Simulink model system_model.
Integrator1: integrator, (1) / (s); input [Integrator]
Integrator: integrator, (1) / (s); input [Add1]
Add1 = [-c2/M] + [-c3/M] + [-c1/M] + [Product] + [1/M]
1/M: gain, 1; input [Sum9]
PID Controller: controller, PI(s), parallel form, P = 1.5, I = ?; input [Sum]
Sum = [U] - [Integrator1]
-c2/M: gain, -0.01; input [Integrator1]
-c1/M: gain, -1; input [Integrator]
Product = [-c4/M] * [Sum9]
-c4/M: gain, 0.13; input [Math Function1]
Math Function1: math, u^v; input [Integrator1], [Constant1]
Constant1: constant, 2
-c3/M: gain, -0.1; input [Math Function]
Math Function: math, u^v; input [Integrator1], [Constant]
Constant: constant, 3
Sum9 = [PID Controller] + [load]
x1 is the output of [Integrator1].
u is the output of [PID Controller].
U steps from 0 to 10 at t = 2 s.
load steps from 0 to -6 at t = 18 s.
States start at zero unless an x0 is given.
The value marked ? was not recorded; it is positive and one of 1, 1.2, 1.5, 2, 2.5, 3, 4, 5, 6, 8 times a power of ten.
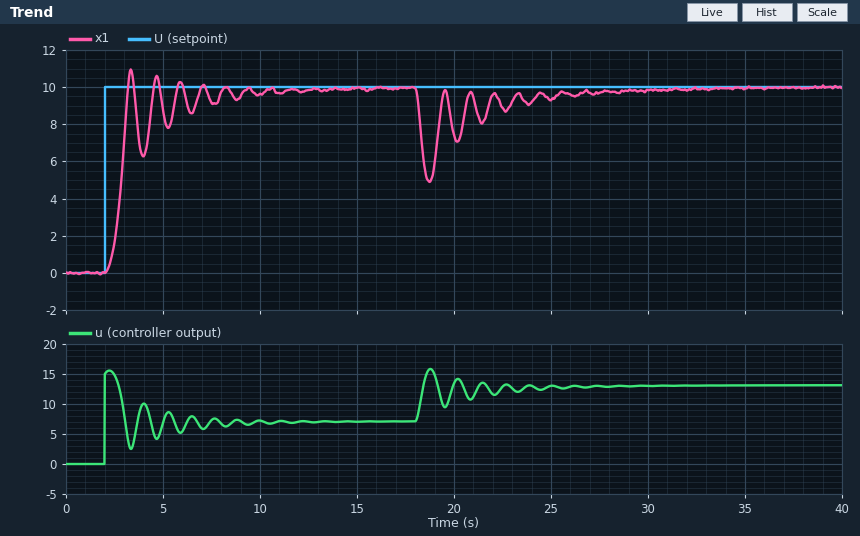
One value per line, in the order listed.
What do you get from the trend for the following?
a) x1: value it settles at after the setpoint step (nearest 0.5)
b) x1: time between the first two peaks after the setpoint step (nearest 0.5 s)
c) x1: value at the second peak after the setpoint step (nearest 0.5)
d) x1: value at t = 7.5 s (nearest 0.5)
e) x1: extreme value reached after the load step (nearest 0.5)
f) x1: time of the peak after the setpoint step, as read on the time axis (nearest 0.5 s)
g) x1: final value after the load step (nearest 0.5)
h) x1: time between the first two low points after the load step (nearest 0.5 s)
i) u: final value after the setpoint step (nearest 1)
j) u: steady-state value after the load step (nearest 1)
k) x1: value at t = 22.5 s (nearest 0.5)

10.0
1.5 s
10.5
9.0
5.0
3.5 s
10.0
1.5 s
7
13
9.0
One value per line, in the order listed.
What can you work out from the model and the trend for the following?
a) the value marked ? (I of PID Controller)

0.5
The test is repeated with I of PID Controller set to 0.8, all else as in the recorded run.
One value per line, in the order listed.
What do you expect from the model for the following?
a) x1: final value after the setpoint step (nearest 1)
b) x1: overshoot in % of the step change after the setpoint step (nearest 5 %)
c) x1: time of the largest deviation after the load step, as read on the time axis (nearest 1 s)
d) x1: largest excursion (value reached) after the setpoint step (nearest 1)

10
20 %
19 s
12
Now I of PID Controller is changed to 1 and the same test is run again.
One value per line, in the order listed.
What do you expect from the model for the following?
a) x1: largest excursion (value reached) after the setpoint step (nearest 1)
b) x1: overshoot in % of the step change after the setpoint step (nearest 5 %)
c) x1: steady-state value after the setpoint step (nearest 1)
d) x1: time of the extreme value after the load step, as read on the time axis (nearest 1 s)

13
30 %
10
19 s
